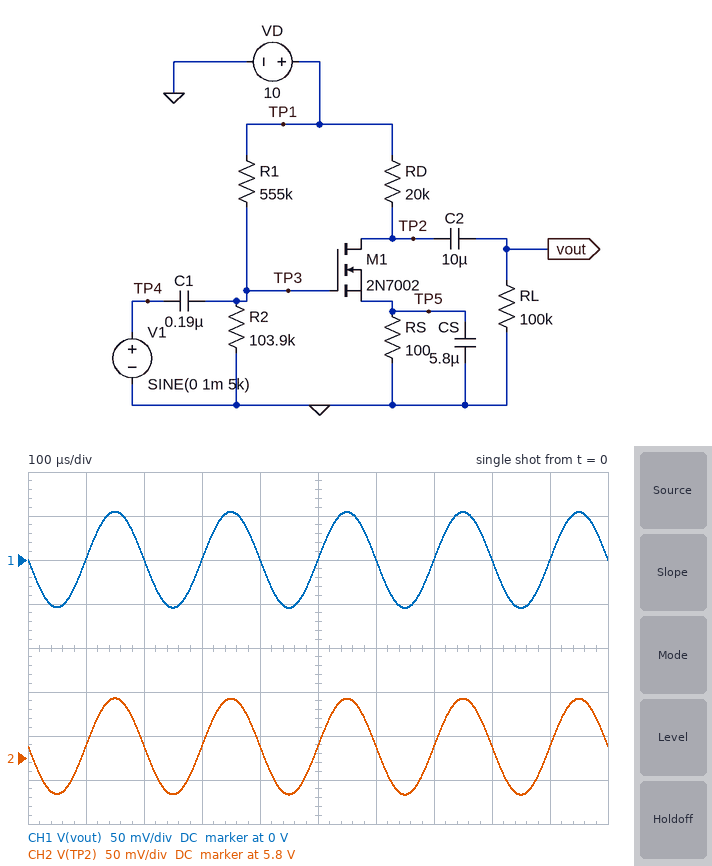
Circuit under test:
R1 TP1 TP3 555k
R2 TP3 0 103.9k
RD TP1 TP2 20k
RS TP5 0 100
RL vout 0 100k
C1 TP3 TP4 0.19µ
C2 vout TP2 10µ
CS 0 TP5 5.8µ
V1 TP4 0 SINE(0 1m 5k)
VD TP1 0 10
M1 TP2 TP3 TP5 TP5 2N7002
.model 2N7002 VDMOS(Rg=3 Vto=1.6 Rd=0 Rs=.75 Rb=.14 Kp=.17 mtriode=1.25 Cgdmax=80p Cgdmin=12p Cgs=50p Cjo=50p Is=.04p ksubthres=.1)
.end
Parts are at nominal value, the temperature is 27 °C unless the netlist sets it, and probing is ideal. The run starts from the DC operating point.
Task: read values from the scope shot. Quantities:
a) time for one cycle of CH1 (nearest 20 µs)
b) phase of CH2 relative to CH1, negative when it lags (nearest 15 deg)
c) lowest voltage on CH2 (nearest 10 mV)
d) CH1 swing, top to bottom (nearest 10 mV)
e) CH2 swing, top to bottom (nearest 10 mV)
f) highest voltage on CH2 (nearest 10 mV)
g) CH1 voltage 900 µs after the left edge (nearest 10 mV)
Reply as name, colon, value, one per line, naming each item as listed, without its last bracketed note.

time for one cycle of CH1: 200 µs
phase of CH2 relative to CH1, negative when it lags: 0 deg
lowest voltage on CH2: 5.76 V
CH1 swing, top to bottom: 110 mV
CH2 swing, top to bottom: 110 mV
highest voltage on CH2: 5.87 V
CH1 voltage 900 µs after the left edge: 0 V
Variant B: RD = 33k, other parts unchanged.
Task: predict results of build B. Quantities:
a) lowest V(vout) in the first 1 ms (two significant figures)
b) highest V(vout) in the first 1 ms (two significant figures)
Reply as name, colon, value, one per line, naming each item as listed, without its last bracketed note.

lowest V(vout) in the first 1 ms: -81 mV
highest V(vout) in the first 1 ms: 81 mV
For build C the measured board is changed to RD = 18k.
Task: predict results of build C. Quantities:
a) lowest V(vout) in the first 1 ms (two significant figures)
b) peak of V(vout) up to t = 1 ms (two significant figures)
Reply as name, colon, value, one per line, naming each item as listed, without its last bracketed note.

lowest V(vout) in the first 1 ms: -50 mV
peak of V(vout) up to t = 1 ms: 50 mV
